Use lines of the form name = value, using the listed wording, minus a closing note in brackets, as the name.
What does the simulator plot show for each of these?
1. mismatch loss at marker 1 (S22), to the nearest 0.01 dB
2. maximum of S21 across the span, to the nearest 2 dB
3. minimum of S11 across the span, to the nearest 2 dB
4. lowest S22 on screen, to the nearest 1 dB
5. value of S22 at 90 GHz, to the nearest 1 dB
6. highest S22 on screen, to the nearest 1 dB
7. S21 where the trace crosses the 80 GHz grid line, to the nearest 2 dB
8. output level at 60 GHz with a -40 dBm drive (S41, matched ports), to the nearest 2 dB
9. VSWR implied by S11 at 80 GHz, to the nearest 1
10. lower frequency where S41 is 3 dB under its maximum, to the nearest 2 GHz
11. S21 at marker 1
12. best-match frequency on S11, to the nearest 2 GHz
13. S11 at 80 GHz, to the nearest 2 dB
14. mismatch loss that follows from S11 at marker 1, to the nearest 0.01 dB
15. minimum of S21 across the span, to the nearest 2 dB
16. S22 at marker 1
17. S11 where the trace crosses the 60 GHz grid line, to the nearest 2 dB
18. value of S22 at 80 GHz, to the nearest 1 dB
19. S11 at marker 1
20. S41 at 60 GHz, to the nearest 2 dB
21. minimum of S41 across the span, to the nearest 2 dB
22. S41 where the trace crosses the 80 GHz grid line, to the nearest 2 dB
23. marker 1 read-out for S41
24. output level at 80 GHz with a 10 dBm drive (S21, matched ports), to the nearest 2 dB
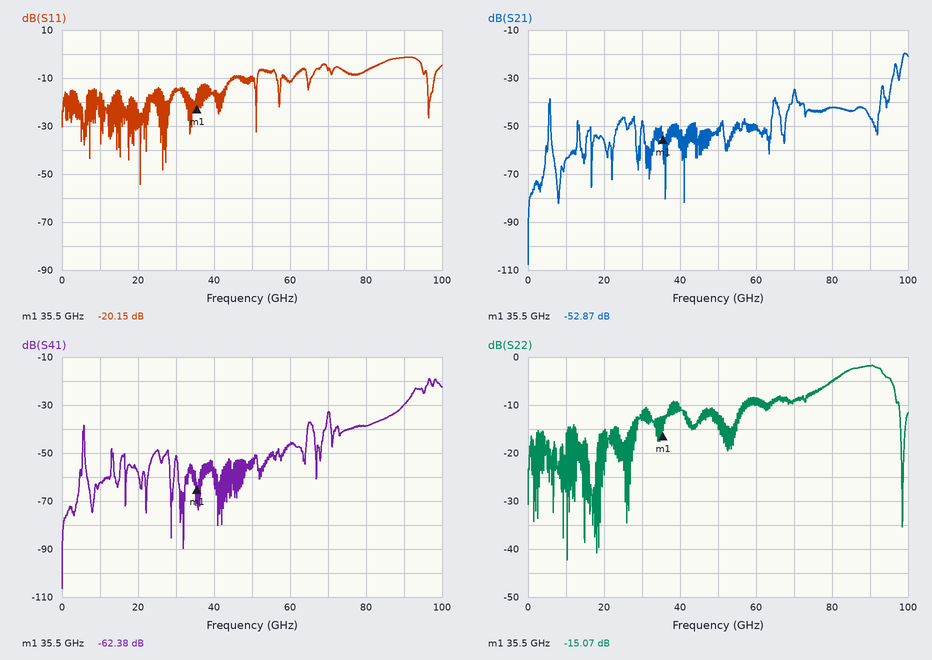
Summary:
mismatch loss at marker 1 (S22), to the nearest 0.01 dB = 0.14 dB
maximum of S21 across the span, to the nearest 2 dB = -20 dB
minimum of S11 across the span, to the nearest 2 dB = -54 dB
lowest S22 on screen, to the nearest 1 dB = -42 dB
value of S22 at 90 GHz, to the nearest 1 dB = -2 dB
highest S22 on screen, to the nearest 1 dB = -2 dB
S21 where the trace crosses the 80 GHz grid line, to the nearest 2 dB = -42 dB
output level at 60 GHz with a -40 dBm drive (S41, matched ports), to the nearest 2 dB = -86 dBm
VSWR implied by S11 at 80 GHz, to the nearest 1 = 3
lower frequency where S41 is 3 dB under its maximum, to the nearest 2 GHz = 96 GHz
S21 at marker 1 = -52.87 dB
best-match frequency on S11, to the nearest 2 GHz = 20 GHz
S11 at 80 GHz, to the nearest 2 dB = -6 dB
mismatch loss that follows from S11 at marker 1, to the nearest 0.01 dB = 0.04 dB
minimum of S21 across the span, to the nearest 2 dB = -108 dB
S22 at marker 1 = -15.07 dB
S11 where the trace crosses the 60 GHz grid line, to the nearest 2 dB = -12 dB
value of S22 at 80 GHz, to the nearest 1 dB = -5 dB
S11 at marker 1 = -20.15 dB
S41 at 60 GHz, to the nearest 2 dB = -46 dB
minimum of S41 across the span, to the nearest 2 dB = -106 dB
S41 where the trace crosses the 80 GHz grid line, to the nearest 2 dB = -38 dB
marker 1 read-out for S41 = -62.38 dB
output level at 80 GHz with a 10 dBm drive (S21, matched ports), to the nearest 2 dB = -32 dBm
